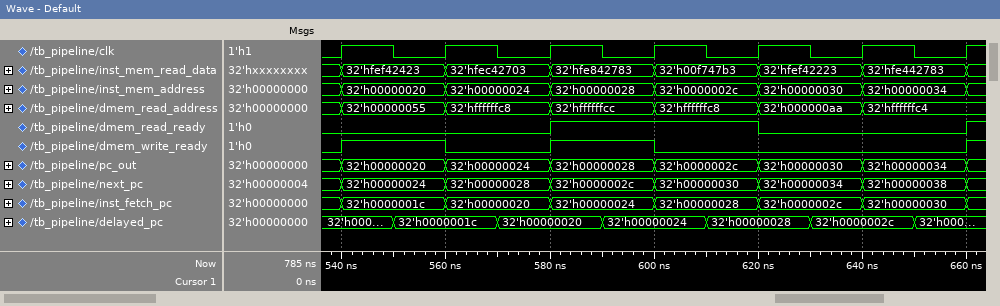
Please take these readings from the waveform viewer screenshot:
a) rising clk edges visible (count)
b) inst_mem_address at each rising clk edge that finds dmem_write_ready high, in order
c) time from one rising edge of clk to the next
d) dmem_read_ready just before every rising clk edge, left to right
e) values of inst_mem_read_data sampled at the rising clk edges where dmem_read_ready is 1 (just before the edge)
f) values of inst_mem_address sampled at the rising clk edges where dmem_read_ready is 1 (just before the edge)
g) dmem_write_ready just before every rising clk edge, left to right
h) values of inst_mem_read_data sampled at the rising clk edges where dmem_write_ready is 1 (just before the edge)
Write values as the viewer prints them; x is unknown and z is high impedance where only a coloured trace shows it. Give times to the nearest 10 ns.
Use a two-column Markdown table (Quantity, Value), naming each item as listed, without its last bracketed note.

| Quantity | Value |
|---|---|
| rising clk edges visible | 7 |
| inst_mem_address at each rising clk edge that finds dmem_write_ready high, in order | 32'h00000020, 32'h00000028 |
| time from one rising edge of clk to the next | 20 ns |
| dmem_read_ready just before every rising clk edge, left to right | 0 0 0 1 1 0 0 |
| values of inst_mem_read_data sampled at the rising clk edges where dmem_read_ready is 1 | 32'hfe842783, 32'h00f747b3 |
| values of inst_mem_address sampled at the rising clk edges where dmem_read_ready is 1 | 32'h00000028, 32'h0000002c |
| dmem_write_ready just before every rising clk edge, left to right | 0 1 0 1 0 0 0 |
| values of inst_mem_read_data sampled at the rising clk edges where dmem_write_ready is 1 | 32'hfef42423, 32'hfe842783 |
